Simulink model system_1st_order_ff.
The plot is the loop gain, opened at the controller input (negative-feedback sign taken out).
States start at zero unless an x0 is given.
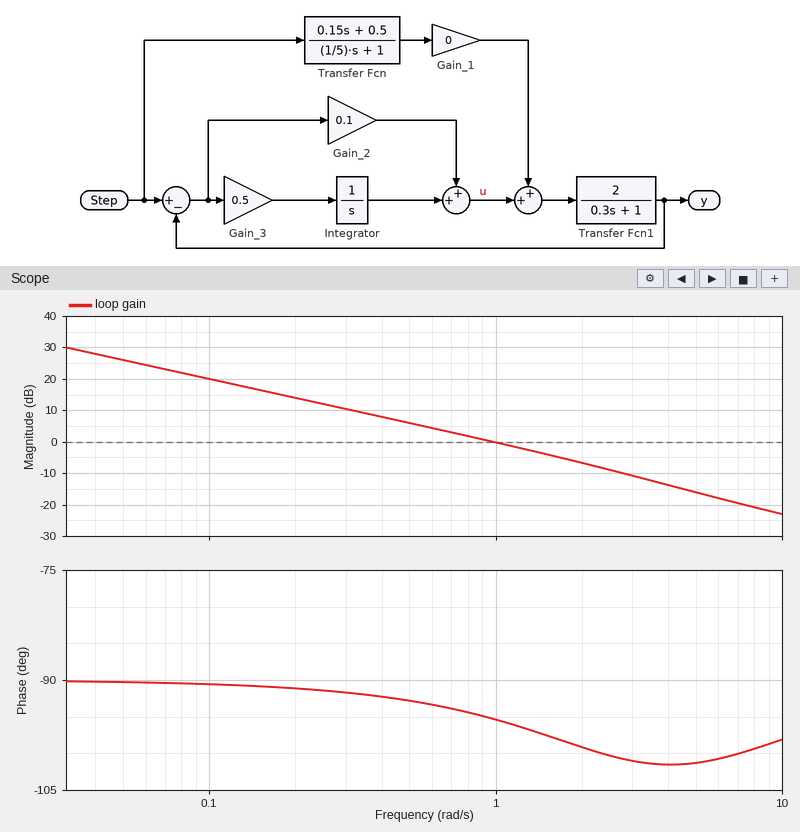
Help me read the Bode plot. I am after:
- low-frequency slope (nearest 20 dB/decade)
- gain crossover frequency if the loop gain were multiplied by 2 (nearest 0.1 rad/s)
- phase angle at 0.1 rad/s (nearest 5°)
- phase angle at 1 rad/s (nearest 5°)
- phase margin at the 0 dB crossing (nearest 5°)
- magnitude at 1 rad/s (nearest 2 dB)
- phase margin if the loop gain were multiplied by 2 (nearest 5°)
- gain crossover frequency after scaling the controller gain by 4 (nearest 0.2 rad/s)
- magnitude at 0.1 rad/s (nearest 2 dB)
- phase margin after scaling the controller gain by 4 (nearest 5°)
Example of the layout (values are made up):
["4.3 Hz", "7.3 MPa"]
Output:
["-20 dB/decade", "1.9 rad/s", "-90°", "-95°", "85°", "0 dB", "80°", "3.4 rad/s", "20 dB", "80°"]
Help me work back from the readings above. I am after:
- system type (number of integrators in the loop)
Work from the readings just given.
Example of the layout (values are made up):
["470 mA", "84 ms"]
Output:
["1"]
